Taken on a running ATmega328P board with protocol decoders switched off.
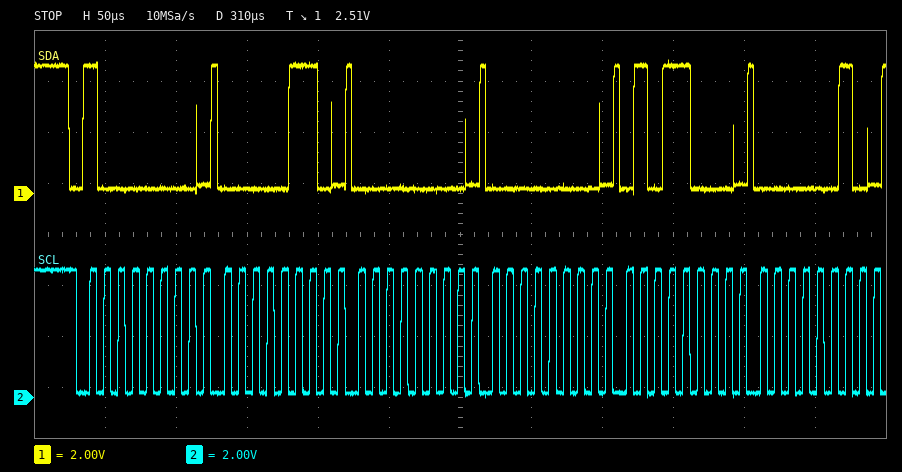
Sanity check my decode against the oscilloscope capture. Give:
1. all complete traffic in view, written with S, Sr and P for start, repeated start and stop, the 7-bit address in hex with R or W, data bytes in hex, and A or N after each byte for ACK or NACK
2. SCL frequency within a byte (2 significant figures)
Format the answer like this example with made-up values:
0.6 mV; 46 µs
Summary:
S 40W A 06 A 00 A 00 A 58 A 02 A; 100 kHz
